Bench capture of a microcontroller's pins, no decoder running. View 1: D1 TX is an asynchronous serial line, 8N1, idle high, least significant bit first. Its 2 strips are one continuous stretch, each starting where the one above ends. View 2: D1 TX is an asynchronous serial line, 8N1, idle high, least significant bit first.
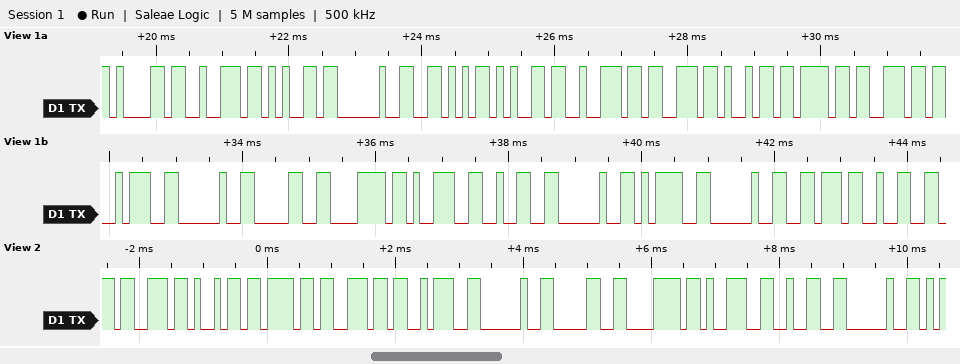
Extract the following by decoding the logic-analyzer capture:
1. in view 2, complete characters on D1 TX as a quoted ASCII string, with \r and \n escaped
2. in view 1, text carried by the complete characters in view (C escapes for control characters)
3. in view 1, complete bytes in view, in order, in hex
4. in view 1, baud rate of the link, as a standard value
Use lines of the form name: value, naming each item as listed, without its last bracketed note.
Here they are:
in view 2, complete characters on D1 TX as a quoted ASCII string, with \r and \n escaped: "sion: 0x92 "
in view 1, text carried by the complete characters in view: "are Version: 0x92 = v2"
in view 1, complete bytes in view, in order, in hex: 61 72 65 20 56 65 72 73 69 6F 6E 3A 20 30 78 39 32 20 3D 20 76 32
in view 1, baud rate of the link, as a standard value: 9600 baud
